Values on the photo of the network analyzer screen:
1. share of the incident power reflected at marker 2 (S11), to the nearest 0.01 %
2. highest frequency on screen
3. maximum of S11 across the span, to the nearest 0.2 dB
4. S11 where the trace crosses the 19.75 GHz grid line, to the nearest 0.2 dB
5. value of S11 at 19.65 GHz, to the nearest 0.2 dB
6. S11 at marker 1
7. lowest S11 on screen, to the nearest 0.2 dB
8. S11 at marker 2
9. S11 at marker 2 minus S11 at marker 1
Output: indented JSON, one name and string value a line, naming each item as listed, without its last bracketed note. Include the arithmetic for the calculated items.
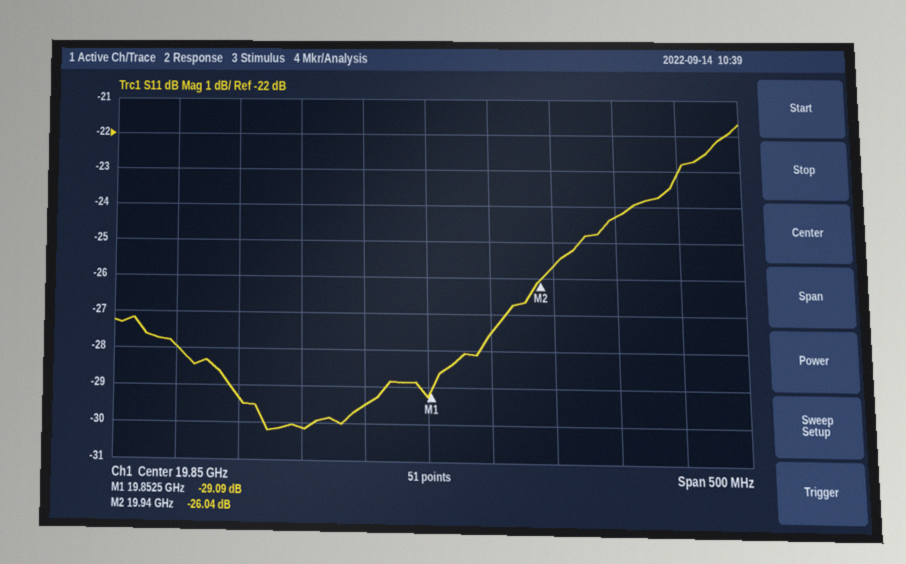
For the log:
{
  "share of the incident power reflected at marker 2 (S11), to the nearest 0.01 %": "10^(-26.04/10) ≈ 0.25 %",
  "highest frequency on screen": "20.1 GHz",
  "maximum of S11 across the span, to the nearest 0.2 dB": "-21.6 dB",
  "S11 where the trace crosses the 19.75 GHz grid line, to the nearest 0.2 dB": "-30.2 dB",
  "value of S11 at 19.65 GHz, to the nearest 0.2 dB": "-28.0 dB",
  "S11 at marker 1": "-29.09 dB",
  "lowest S11 on screen, to the nearest 0.2 dB": "-30.2 dB",
  "S11 at marker 2": "-26.04 dB",
  "S11 at marker 2 minus S11 at marker 1": "-26.04 − (-29.09) = 3.05 dB"
}
